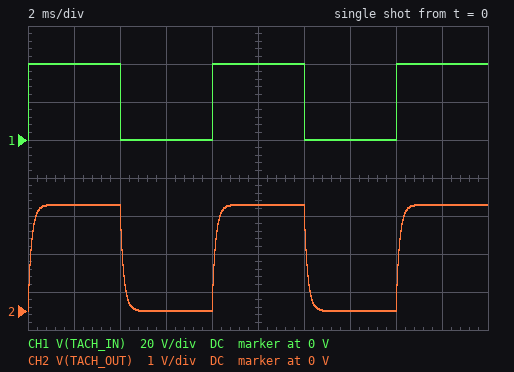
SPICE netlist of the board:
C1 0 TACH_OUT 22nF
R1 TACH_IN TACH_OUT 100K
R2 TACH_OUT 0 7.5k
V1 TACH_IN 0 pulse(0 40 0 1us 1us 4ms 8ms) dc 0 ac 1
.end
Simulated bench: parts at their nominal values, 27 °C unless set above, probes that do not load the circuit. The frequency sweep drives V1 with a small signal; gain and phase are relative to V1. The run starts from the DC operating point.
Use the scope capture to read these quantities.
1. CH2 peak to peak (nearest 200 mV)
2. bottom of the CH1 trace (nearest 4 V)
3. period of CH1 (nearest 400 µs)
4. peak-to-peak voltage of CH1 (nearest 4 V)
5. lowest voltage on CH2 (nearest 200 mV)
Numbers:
2.8 V
0 V
8.0 ms
40 V
0 V
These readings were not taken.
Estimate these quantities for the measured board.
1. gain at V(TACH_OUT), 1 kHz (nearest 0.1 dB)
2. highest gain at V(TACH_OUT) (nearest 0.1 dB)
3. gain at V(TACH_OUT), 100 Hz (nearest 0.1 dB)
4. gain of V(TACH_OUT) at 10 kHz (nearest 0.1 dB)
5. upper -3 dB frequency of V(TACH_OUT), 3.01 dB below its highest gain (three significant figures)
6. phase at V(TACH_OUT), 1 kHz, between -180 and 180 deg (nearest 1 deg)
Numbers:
-26.0 dB
-23.1 dB
-23.2 dB
-42.9 dB
1.04 kHz
-44 deg
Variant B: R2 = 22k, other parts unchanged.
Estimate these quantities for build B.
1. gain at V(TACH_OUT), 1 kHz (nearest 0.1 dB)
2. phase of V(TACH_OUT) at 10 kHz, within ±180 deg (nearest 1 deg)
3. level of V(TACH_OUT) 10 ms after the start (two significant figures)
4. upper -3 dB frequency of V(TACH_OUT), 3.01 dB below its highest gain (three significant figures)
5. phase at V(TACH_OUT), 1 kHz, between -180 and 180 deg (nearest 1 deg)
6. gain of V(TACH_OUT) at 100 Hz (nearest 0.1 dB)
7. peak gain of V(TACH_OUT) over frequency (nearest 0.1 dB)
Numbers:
-23.5 dB
-88 deg
7.2 V
401 Hz
-68 deg
-15.1 dB
-14.9 dB
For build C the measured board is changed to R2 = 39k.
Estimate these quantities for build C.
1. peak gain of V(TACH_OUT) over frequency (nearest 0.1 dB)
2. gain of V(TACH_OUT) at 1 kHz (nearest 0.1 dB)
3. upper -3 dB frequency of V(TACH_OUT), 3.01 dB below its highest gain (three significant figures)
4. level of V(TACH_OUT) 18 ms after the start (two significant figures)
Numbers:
-11.0 dB
-23.1 dB
258 Hz
11 V
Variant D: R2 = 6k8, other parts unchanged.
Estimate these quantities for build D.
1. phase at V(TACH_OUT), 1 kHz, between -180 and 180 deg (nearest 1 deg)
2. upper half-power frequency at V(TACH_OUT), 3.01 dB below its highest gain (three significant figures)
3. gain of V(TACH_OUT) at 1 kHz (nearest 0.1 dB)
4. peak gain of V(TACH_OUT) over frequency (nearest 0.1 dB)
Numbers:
-41 deg
1.14 kHz
-26.4 dB
-23.9 dB
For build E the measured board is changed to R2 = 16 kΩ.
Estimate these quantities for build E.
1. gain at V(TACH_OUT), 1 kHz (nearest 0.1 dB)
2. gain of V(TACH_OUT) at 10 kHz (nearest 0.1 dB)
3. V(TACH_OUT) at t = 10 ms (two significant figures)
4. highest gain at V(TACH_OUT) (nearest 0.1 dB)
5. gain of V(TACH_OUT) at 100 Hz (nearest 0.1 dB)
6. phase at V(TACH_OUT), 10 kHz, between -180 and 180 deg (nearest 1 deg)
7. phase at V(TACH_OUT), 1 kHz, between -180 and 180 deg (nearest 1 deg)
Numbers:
-23.9 dB
-42.8 dB
5.5 V
-17.2 dB
-17.4 dB
-87 deg
-62 deg
